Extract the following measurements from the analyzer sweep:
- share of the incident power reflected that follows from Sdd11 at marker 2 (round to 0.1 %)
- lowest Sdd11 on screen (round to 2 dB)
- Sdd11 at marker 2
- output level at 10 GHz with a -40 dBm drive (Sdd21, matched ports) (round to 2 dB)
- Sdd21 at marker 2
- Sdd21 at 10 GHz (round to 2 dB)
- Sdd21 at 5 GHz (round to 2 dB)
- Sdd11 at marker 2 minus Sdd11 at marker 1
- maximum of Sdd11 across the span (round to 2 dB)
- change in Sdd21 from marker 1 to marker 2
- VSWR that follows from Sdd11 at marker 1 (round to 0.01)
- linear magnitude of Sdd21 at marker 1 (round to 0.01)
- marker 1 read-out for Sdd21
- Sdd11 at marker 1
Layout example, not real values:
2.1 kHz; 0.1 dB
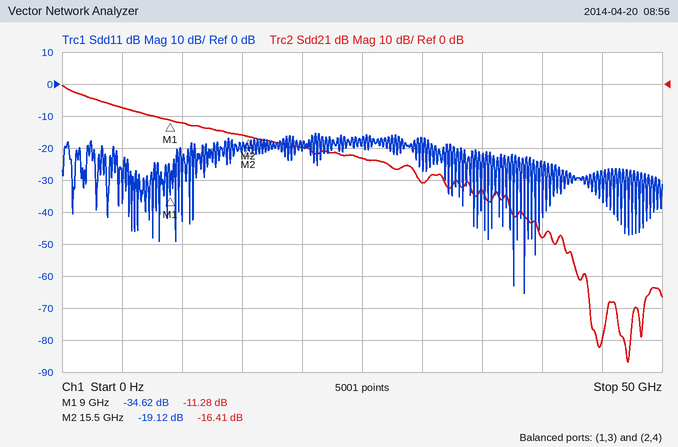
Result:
1.2 %; -66 dB; -19.12 dB; -52 dBm; -16.41 dB; -12 dB; -8 dB; 15.50 dB; -16 dB; -5.13 dB; 1.04; 0.27; -11.28 dB; -34.62 dB
